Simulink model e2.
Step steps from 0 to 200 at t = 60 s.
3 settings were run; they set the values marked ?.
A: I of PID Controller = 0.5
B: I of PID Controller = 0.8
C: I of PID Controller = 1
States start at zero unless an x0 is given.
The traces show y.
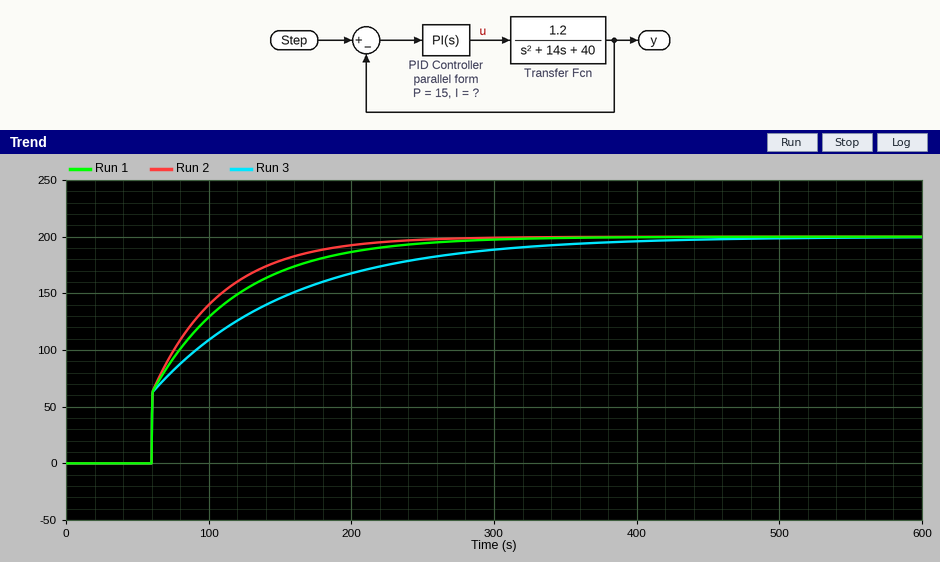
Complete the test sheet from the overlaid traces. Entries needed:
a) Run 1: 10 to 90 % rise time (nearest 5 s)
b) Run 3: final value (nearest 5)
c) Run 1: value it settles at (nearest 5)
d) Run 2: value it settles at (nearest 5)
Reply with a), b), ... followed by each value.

a) 115 s
b) 200
c) 200
d) 200
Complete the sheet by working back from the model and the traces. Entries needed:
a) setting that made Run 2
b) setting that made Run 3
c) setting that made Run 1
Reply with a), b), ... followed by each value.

a) C
b) A
c) B
